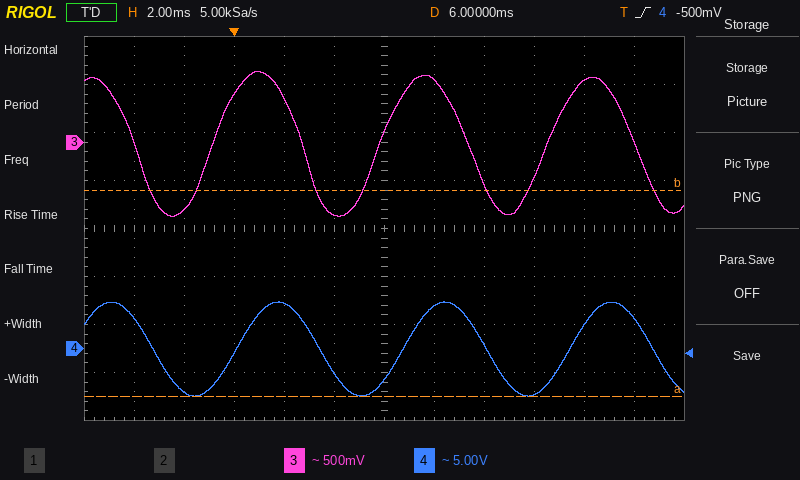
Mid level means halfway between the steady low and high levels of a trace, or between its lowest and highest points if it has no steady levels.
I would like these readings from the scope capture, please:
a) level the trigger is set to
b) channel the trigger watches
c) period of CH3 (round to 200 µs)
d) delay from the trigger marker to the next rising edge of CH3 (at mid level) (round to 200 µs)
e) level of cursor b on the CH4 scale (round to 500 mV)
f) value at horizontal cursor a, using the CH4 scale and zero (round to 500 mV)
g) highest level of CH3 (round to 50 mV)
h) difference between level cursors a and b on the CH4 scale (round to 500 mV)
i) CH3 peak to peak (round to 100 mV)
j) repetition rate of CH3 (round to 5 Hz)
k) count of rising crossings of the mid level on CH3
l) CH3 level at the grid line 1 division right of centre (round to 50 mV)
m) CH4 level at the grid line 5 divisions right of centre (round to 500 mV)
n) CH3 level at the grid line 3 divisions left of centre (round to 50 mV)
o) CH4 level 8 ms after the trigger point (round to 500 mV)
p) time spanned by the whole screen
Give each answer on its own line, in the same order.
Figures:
-500 mV
CH4
6.6 ms
5.8 ms
16.5 V
-5.0 V
750 mV
21.5 V
1.50 V
150 Hz
3
650 mV
3.0 V
500 mV
4.5 V
24 ms
